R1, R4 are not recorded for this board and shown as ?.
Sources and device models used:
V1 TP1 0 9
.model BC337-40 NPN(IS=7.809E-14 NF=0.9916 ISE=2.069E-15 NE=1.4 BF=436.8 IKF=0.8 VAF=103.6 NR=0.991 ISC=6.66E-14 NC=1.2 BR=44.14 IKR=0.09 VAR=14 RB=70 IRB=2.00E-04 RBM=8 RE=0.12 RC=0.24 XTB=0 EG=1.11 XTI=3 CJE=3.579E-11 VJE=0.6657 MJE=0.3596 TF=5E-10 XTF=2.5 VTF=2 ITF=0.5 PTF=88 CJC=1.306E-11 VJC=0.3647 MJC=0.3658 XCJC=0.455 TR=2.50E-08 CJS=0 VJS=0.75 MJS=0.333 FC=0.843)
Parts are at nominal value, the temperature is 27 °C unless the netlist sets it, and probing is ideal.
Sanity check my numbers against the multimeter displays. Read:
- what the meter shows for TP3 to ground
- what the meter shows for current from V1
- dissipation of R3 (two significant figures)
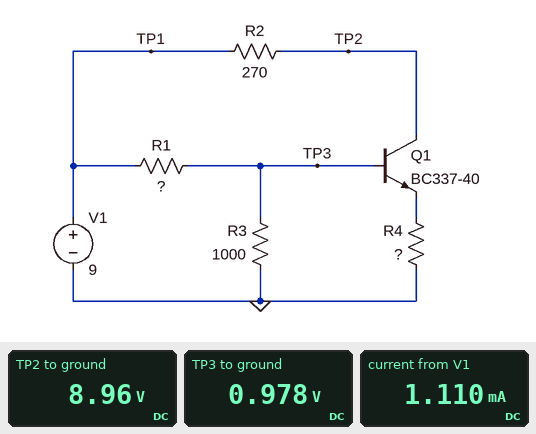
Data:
0.978 V
1.110 mA
960 µW
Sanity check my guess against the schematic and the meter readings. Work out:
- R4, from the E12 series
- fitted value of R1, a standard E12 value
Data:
3.3 kΩ
8.2 kΩ
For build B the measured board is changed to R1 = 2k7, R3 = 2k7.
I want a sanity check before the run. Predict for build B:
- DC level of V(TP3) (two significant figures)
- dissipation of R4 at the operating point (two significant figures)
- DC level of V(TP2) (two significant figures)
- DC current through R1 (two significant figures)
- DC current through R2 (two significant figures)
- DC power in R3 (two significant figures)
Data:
4.5 V
4.6 mW
8.7 V
1.7 mA
1.2 mA
7.5 mW
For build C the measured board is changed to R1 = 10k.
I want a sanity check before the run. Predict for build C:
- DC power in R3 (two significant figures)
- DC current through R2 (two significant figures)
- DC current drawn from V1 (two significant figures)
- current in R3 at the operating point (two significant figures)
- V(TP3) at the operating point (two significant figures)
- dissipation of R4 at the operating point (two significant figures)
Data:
670 µW
86 µA
900 µA
820 µA
820 mV
25 µW
